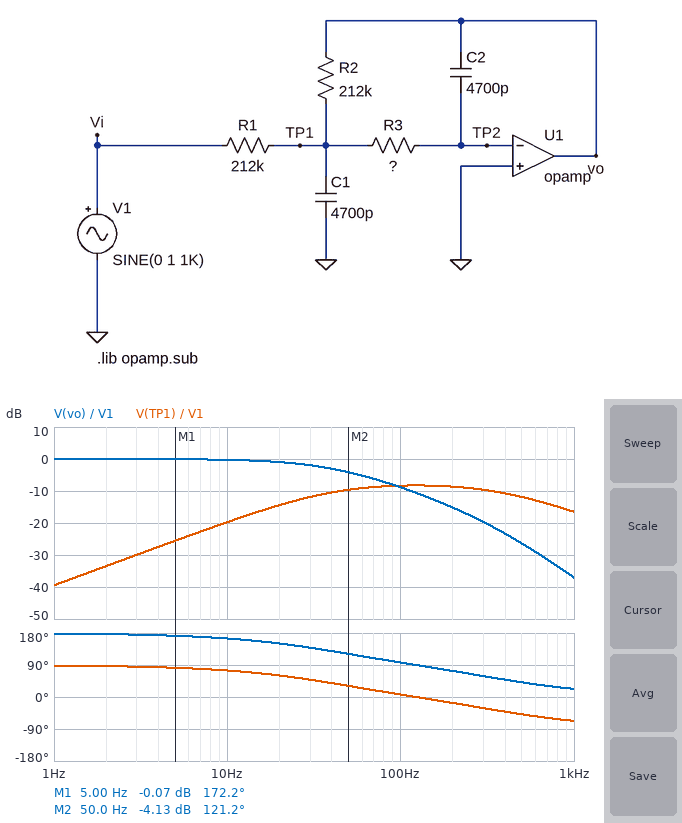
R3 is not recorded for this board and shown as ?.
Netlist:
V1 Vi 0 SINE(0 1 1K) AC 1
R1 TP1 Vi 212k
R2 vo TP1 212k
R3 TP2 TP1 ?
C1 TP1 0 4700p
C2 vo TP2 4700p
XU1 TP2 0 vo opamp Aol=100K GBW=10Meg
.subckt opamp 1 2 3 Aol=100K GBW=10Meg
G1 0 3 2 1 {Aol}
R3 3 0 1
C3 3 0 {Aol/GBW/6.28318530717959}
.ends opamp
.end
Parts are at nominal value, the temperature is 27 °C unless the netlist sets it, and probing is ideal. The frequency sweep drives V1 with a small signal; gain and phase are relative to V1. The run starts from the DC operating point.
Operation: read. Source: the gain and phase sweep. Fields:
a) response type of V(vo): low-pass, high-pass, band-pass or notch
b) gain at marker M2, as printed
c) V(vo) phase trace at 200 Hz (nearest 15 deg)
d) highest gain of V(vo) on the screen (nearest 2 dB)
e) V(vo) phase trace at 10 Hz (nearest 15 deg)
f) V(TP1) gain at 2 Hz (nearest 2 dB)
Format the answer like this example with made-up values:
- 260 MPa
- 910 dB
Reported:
- low-pass
- -4.13 dB
- 75 deg
- 0 dB
- 165 deg
- -34 dB
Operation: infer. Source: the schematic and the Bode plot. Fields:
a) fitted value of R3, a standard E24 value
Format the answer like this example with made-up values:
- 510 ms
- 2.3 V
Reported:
- 360 kΩ
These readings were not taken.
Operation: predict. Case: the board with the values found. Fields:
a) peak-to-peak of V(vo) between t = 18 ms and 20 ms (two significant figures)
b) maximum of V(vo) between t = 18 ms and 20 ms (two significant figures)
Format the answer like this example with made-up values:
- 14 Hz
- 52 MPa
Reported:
- 28 mV
- 14 mV
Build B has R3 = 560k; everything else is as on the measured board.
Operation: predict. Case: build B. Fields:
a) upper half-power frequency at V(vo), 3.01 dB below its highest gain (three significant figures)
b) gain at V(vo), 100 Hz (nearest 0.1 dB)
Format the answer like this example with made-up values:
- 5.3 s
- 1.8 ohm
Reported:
- 27.2 Hz
- -11.9 dB
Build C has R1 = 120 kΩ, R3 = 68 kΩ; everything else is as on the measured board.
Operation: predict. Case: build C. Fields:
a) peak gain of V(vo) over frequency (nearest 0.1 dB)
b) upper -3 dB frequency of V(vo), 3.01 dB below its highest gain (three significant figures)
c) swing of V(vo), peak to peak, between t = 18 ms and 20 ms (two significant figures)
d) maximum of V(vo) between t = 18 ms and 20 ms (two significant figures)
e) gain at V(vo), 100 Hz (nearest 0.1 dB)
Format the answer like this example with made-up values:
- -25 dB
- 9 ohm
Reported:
- 4.9 dB
- 92.9 Hz
- 210 mV
- 110 mV
- 1.6 dB
